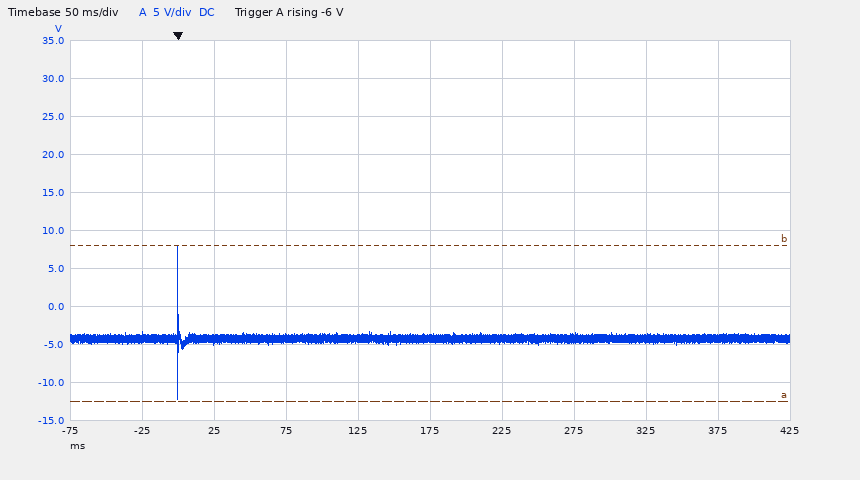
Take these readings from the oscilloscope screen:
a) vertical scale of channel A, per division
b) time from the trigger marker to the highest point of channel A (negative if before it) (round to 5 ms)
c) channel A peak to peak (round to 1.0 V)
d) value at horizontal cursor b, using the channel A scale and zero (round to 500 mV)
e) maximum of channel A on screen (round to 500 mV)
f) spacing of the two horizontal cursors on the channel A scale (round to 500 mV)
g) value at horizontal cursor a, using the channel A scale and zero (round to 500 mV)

5 V
0 ms
20.0 V
8.0 V
8.0 V
20.5 V
-12.5 V
